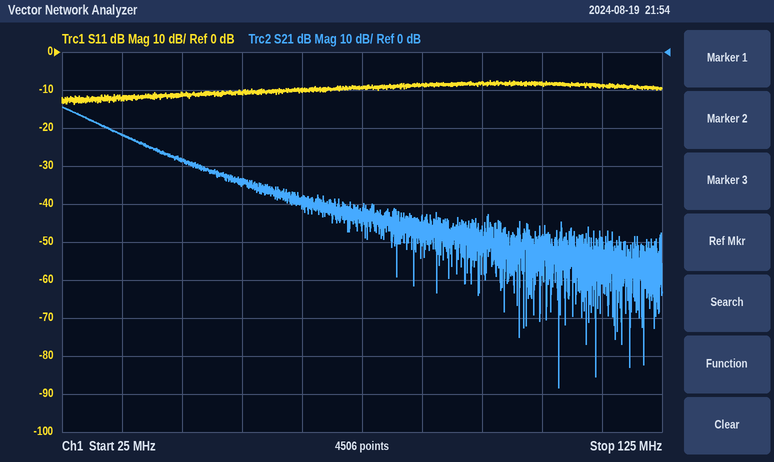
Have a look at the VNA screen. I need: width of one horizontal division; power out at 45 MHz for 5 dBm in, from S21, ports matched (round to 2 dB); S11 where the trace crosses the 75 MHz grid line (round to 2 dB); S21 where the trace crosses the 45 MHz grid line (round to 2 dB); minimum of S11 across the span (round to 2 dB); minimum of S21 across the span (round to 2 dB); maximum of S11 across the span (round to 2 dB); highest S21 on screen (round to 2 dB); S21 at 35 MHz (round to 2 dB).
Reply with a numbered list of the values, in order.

1. 10 MHz
2. -24 dBm
3. -10 dB
4. -28 dB
5. -14 dB
6. -88 dB
7. -8 dB
8. -14 dB
9. -22 dB
